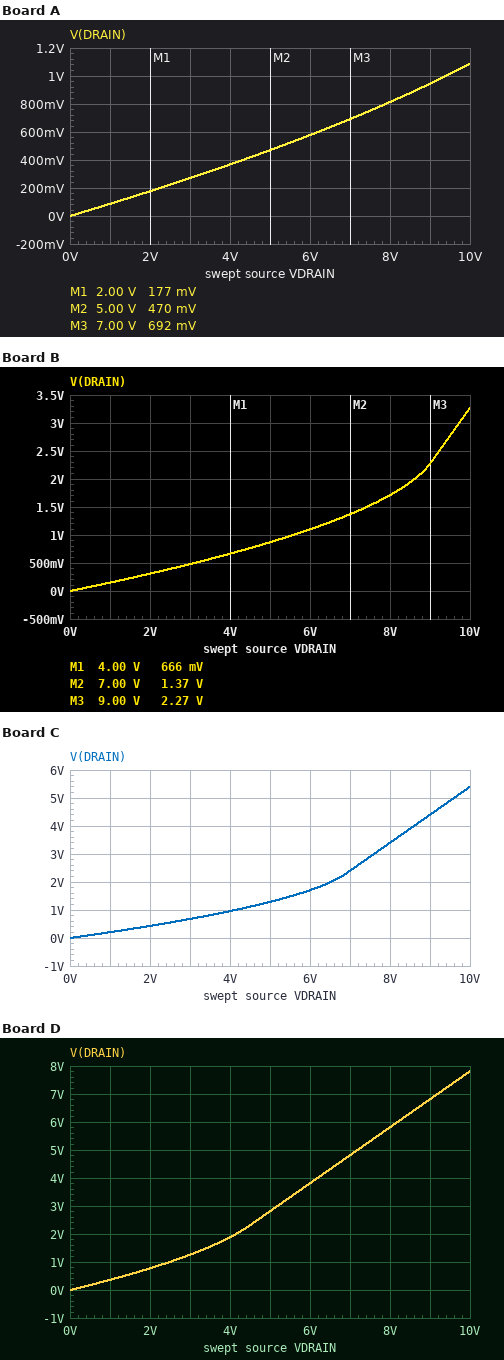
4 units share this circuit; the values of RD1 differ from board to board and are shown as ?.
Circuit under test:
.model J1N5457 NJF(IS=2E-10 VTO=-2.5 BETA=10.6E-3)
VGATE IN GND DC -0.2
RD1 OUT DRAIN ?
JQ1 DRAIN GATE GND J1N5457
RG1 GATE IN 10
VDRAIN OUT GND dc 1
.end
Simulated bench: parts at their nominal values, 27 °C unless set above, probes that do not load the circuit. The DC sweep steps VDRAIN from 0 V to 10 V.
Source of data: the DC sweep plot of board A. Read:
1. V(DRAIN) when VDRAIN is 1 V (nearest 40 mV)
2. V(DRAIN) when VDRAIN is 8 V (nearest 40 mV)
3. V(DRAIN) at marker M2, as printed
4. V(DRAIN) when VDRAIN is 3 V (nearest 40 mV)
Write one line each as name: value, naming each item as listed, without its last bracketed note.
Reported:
V(DRAIN) when VDRAIN is 1 V: 80 mV
V(DRAIN) when VDRAIN is 8 V: 800 mV
V(DRAIN) at marker M2, as printed: 470 mV
V(DRAIN) when VDRAIN is 3 V: 280 mV
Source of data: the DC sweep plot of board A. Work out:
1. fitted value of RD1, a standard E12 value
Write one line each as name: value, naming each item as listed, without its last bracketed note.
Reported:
fitted value of RD1, a standard E12 value: 220 Ω
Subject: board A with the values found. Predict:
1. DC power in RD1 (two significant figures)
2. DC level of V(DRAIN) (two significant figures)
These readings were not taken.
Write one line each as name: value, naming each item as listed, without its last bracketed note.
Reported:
DC power in RD1: 3.8 mW
DC level of V(DRAIN): 87 mV
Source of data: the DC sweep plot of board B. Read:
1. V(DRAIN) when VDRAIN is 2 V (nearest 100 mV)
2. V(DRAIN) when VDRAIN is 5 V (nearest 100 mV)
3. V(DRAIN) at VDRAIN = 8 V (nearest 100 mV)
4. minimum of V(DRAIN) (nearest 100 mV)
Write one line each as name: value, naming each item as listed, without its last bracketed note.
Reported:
V(DRAIN) when VDRAIN is 2 V: 300 mV
V(DRAIN) when VDRAIN is 5 V: 900 mV
V(DRAIN) at VDRAIN = 8 V: 1.7 V
minimum of V(DRAIN): 0 V
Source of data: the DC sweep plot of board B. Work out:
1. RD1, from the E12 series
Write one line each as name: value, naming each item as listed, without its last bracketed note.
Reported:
RD1, from the E12 series: 120 Ω
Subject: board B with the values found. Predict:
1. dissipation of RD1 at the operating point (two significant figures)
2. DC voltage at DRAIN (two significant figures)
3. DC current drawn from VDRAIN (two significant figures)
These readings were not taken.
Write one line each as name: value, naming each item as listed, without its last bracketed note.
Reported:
dissipation of RD1 at the operating point: 6.0 mW
DC voltage at DRAIN: 150 mV
DC current drawn from VDRAIN: 7.1 mA
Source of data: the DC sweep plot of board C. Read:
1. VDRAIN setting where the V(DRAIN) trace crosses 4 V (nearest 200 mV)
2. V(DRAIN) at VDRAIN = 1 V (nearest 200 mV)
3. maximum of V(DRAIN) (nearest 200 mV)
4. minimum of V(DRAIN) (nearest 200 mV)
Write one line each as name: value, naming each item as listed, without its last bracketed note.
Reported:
VDRAIN setting where the V(DRAIN) trace crosses 4 V: 8.6 V
V(DRAIN) at VDRAIN = 1 V: 200 mV
maximum of V(DRAIN): 5.4 V
minimum of V(DRAIN): 0 V
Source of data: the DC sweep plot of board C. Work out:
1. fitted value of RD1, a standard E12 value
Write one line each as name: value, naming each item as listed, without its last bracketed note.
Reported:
fitted value of RD1, a standard E12 value: 82 Ω
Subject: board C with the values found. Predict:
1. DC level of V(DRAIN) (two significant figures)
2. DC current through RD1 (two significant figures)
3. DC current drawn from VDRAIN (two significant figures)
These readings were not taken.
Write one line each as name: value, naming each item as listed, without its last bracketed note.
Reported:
DC level of V(DRAIN): 210 mV
DC current through RD1: 9.7 mA
DC current drawn from VDRAIN: 9.7 mA
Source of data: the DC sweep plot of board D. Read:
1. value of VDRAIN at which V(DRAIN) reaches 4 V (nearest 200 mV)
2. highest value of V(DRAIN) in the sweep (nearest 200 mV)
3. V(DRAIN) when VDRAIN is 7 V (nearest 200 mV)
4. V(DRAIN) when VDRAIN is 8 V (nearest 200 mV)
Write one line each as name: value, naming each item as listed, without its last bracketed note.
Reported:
value of VDRAIN at which V(DRAIN) reaches 4 V: 6.2 V
highest value of V(DRAIN) in the sweep: 7.8 V
V(DRAIN) when VDRAIN is 7 V: 4.8 V
V(DRAIN) when VDRAIN is 8 V: 5.8 V
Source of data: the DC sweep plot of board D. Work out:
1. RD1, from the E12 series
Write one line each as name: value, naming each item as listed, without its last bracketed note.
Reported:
RD1, from the E12 series: 39 Ω
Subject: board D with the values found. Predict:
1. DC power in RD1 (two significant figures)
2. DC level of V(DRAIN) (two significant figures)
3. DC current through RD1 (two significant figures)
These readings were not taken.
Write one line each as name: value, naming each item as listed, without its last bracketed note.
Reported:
DC power in RD1: 10 mW
DC level of V(DRAIN): 360 mV
DC current through RD1: 16 mA
